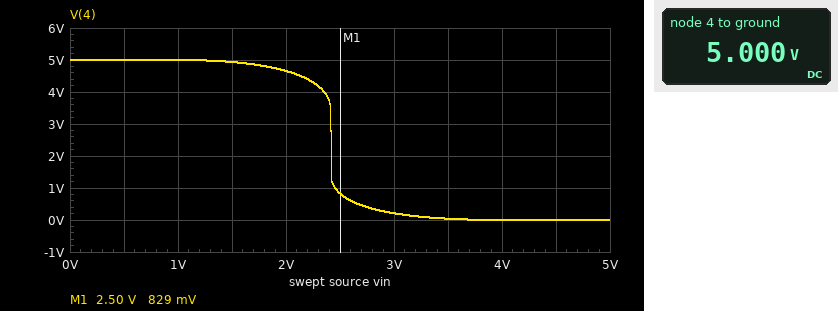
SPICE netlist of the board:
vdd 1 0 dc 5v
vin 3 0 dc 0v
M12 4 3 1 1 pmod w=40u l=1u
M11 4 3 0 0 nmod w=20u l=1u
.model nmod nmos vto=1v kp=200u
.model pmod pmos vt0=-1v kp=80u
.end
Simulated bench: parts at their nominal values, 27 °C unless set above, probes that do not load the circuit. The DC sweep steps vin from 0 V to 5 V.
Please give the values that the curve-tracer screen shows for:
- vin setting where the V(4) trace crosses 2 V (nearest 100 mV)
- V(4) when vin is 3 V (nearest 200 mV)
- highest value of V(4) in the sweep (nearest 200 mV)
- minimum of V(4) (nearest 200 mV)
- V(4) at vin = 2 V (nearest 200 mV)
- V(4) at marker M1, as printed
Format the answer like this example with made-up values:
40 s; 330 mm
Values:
2.4 V; 200 mV; 5.0 V; 0 V; 4.6 V; 829 mV
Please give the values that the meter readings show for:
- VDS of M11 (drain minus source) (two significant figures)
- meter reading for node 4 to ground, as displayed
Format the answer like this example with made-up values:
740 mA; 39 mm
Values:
5.0 V; 5.000 V
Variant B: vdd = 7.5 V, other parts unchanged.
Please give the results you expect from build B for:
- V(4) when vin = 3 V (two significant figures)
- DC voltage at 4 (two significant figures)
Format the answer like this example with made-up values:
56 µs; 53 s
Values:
6.7 V; 7.5 V
